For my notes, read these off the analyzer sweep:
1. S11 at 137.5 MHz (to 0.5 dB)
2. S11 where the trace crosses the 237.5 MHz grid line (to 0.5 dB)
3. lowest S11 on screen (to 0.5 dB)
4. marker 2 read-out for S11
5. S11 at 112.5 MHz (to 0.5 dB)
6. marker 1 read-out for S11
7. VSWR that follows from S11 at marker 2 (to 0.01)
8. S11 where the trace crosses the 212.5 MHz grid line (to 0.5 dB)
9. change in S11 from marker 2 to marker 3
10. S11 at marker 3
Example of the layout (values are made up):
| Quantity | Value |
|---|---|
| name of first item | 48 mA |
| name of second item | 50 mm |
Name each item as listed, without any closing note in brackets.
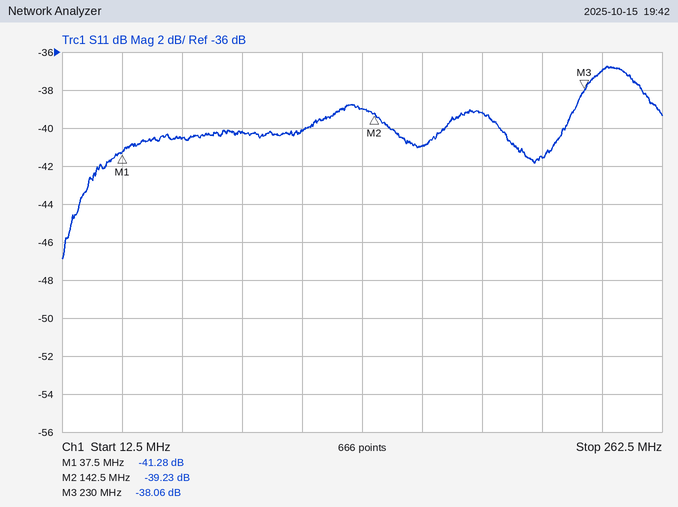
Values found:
| Quantity | Value |
|---|---|
| S11 at 137.5 MHz | -39.0 dB |
| S11 where the trace crosses the 237.5 MHz grid line | -37.0 dB |
| lowest S11 on screen | -47.0 dB |
| marker 2 read-out for S11 | -39.23 dB |
| S11 at 112.5 MHz | -40.0 dB |
| marker 1 read-out for S11 | -41.28 dB |
| VSWR that follows from S11 at marker 2 | 1.02 |
| S11 where the trace crosses the 212.5 MHz grid line | -41.5 dB |
| change in S11 from marker 2 to marker 3 | 1.17 dB |
| S11 at marker 3 | -38.06 dB |
